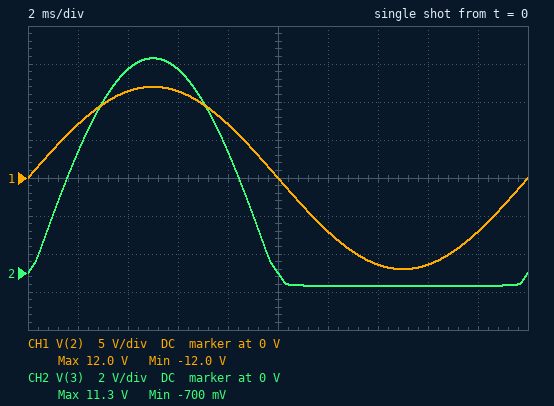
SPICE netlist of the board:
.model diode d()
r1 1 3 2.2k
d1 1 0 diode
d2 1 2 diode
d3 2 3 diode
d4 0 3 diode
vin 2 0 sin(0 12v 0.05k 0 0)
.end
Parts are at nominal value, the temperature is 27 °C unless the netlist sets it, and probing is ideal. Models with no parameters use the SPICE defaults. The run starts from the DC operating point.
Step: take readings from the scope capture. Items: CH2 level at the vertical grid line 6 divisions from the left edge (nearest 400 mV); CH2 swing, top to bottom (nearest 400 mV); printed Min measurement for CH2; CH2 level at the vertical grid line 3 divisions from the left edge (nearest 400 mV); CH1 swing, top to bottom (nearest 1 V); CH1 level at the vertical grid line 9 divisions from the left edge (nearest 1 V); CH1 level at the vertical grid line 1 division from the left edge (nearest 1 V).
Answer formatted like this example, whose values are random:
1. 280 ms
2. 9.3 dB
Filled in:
1. -800 mV
2. 12.0 V
3. -700 mV
4. 10.8 V
5. 24 V
6. -7 V
7. 7 V
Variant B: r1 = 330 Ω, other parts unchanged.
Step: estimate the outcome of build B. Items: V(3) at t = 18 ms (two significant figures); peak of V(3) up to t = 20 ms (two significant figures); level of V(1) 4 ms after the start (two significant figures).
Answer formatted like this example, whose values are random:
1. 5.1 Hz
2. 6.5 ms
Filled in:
1. -730 mV
2. 11 V
3. 740 mV
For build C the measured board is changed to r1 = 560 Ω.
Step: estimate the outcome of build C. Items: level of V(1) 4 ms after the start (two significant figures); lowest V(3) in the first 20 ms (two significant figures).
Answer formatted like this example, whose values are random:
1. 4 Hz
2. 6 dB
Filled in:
1. 730 mV
2. -730 mV
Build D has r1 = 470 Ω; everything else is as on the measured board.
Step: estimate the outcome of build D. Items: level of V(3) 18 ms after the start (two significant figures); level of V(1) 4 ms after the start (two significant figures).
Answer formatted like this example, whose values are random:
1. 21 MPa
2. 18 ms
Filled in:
1. -720 mV
2. 730 mV
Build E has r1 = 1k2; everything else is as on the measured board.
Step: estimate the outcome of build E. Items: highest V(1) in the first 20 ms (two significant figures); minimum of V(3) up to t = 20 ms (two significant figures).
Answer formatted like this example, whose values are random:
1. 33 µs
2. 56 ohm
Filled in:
1. 710 mV
2. -710 mV
